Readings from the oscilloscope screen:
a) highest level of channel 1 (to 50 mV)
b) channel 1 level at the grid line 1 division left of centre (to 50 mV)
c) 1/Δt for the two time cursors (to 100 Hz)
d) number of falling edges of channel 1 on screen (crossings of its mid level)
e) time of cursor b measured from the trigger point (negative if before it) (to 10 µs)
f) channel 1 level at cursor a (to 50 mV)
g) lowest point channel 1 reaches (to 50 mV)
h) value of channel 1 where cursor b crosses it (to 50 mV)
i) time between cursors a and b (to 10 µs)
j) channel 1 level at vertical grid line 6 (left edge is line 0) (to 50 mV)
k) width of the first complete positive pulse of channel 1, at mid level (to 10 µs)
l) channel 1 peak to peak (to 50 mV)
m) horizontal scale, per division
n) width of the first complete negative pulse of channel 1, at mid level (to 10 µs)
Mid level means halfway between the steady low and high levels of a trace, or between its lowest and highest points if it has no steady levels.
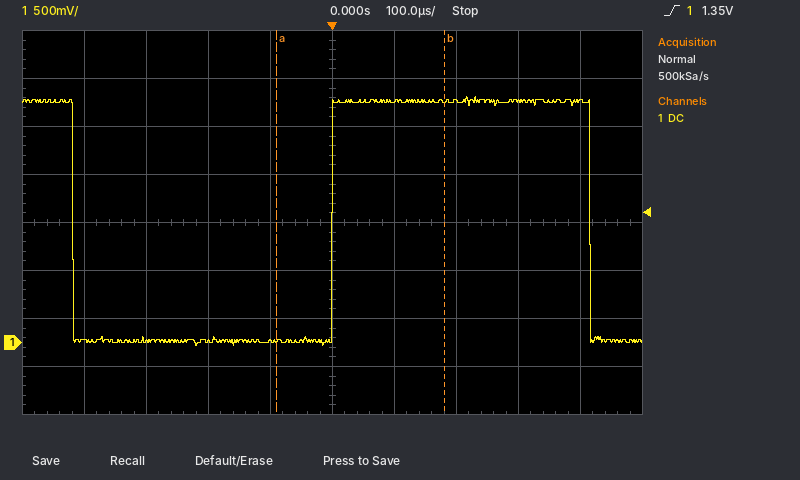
2.55 V
0 mV
3.7 kHz
2
+180 µs
0 mV
-50 mV
2.50 V
270 µs
2.50 V
420 µs
2.60 V
100 µs
420 µs
